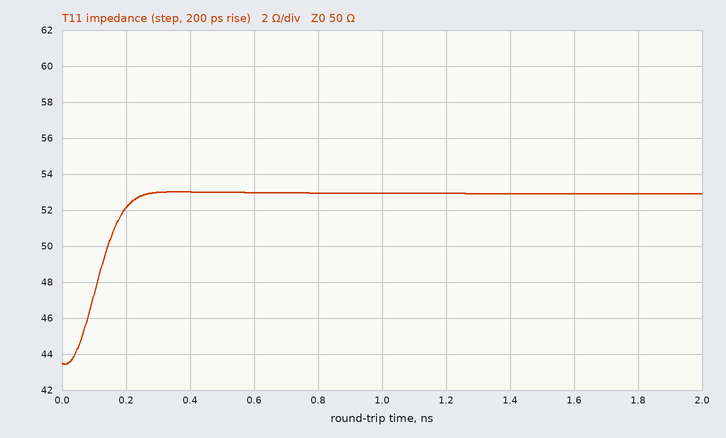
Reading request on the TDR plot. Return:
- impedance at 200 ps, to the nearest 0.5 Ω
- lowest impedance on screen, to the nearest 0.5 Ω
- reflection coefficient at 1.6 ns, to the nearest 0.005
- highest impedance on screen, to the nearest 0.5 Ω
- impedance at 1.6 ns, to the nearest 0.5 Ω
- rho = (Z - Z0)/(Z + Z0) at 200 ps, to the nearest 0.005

52.0 Ω
43.5 Ω
+0.030
53.0 Ω
53.0 Ω
+0.020
